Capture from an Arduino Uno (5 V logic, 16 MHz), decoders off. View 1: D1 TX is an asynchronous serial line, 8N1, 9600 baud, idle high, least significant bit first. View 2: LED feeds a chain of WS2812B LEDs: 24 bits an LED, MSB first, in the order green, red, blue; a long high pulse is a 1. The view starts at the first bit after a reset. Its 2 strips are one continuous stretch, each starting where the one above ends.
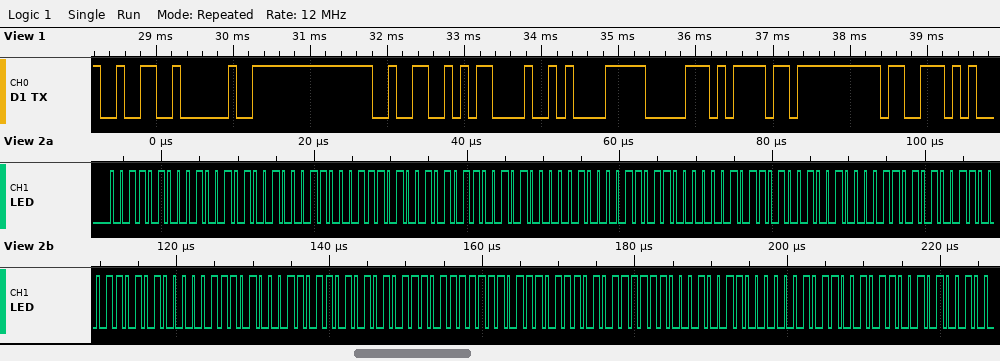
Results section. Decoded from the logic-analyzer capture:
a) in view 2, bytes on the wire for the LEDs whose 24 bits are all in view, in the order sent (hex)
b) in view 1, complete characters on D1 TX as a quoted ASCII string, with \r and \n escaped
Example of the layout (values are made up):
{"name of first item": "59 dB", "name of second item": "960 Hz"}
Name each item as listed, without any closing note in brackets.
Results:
{"in view 2, bytes on the wire for the LEDs whose 24 bits are all in view, in the order sent": "34 4A 46 3A 56 50 43 60 5A 48 6A 63 50 74 6D 57 7F 77 5F 89 81", "in view 1, complete characters on D1 TX as a quoted ASCII string, with \\r and \\n escaped": "\"2 2\\r\\npos\""}
